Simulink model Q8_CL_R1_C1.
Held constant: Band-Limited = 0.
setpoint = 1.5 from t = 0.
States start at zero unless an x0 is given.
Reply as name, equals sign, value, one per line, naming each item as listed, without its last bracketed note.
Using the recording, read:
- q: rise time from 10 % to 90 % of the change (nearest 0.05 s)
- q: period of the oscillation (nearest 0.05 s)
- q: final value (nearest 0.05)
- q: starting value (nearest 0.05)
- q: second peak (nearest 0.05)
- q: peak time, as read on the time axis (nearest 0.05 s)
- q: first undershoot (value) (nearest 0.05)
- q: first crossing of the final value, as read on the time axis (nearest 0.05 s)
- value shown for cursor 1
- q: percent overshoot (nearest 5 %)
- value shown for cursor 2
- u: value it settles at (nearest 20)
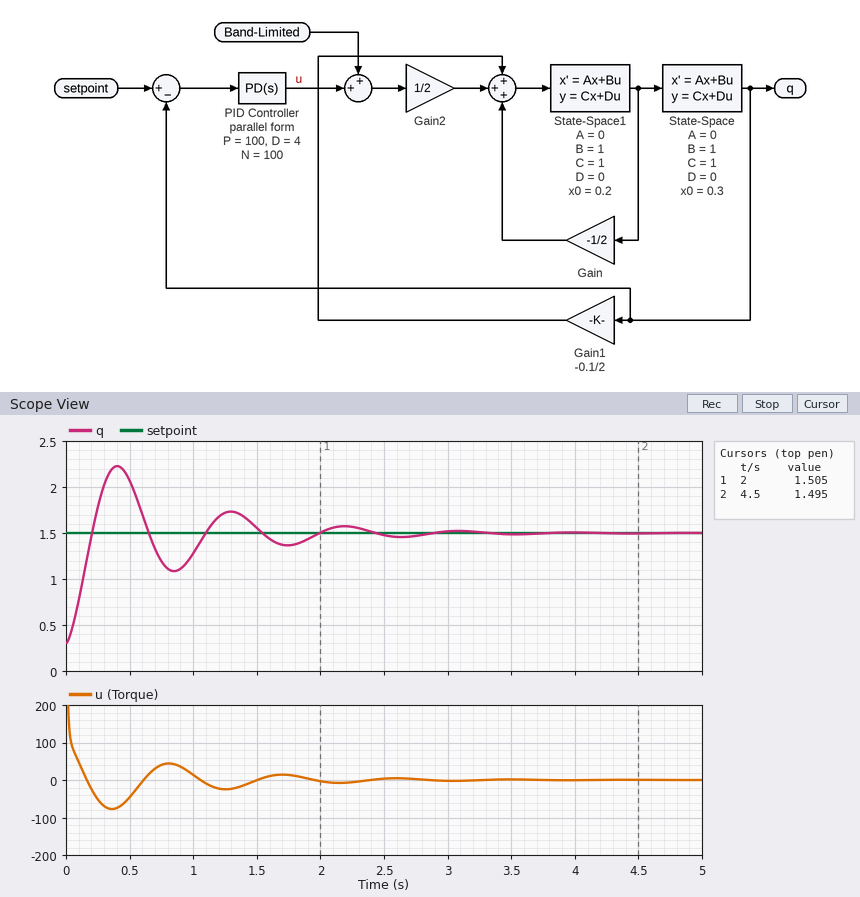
q: rise time from 10 % to 90 % of the change = 0.15 s
q: period of the oscillation = 0.90 s
q: final value = 1.50
q: starting value = 0.30
q: second peak = 1.75
q: peak time, as read on the time axis = 0.40 s
q: first undershoot (value) = 1.10
q: first crossing of the final value, as read on the time axis = 0.20 s
value shown for cursor 1 = 1.505
q: percent overshoot = 60 %
value shown for cursor 2 = 1.495
u: value it settles at = 0
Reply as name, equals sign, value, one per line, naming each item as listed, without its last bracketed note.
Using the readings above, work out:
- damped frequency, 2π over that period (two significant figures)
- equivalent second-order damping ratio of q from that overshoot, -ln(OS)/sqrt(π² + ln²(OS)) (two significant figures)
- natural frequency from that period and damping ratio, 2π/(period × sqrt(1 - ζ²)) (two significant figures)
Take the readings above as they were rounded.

damped frequency, 2π over that period = 7.0 rad/s
equivalent second-order damping ratio of q from that overshoot, -ln(OS)/sqrt(π² + ln²(OS)) = 0.16
natural frequency from that period and damping ratio, 2π/(period × sqrt(1 - ζ²)) = 7.1 rad/s
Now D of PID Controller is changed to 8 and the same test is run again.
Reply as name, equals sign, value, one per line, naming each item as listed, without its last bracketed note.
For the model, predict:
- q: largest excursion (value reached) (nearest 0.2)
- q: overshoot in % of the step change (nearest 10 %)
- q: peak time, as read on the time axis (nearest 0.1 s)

q: largest excursion (value reached) = 2.0
q: overshoot in % of the step change = 40 %
q: peak time, as read on the time axis = 0.4 s
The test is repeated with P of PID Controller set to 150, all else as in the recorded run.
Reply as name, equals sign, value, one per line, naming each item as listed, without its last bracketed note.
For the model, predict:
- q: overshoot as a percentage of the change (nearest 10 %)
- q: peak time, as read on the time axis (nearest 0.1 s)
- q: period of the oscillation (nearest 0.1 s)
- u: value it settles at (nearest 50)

q: overshoot as a percentage of the change = 70 %
q: peak time, as read on the time axis = 0.3 s
q: period of the oscillation = 0.7 s
u: value it settles at = 0
